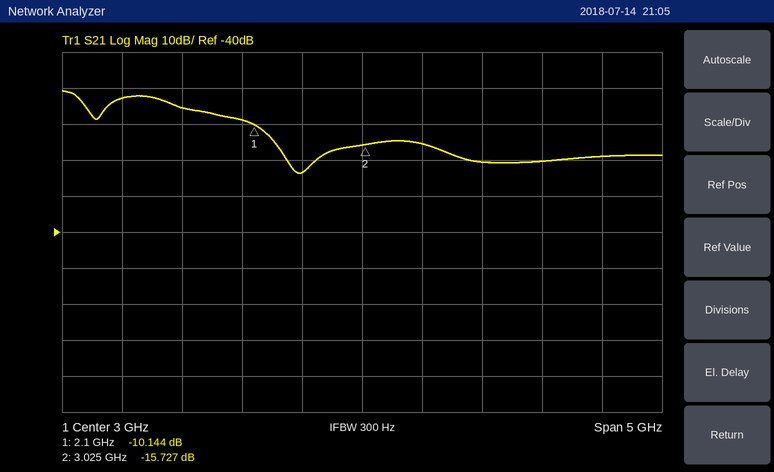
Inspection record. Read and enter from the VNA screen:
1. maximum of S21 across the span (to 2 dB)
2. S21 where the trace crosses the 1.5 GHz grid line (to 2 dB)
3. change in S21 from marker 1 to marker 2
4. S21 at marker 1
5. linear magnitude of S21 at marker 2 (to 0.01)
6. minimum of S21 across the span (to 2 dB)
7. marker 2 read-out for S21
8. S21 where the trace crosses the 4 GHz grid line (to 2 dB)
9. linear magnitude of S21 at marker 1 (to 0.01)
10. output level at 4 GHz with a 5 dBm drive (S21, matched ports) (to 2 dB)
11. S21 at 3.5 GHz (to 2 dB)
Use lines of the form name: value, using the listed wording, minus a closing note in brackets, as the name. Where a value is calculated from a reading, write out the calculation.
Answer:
maximum of S21 across the span: 0 dB
S21 where the trace crosses the 1.5 GHz grid line: -6 dB
change in S21 from marker 1 to marker 2: -15.727 − (-10.144) = -5.583 dB
S21 at marker 1: -10.144 dB
linear magnitude of S21 at marker 2: 10^(-15.727/20) ≈ 0.16
minimum of S21 across the span: -24 dB
marker 2 read-out for S21: -15.727 dB
S21 where the trace crosses the 4 GHz grid line: -20 dB
linear magnitude of S21 at marker 1: 10^(-10.144/20) ≈ 0.31
output level at 4 GHz with a 5 dBm drive (S21, matched ports): 5 dBm + (-20 dB) = -16 dBm
S21 at 3.5 GHz: -16 dB
